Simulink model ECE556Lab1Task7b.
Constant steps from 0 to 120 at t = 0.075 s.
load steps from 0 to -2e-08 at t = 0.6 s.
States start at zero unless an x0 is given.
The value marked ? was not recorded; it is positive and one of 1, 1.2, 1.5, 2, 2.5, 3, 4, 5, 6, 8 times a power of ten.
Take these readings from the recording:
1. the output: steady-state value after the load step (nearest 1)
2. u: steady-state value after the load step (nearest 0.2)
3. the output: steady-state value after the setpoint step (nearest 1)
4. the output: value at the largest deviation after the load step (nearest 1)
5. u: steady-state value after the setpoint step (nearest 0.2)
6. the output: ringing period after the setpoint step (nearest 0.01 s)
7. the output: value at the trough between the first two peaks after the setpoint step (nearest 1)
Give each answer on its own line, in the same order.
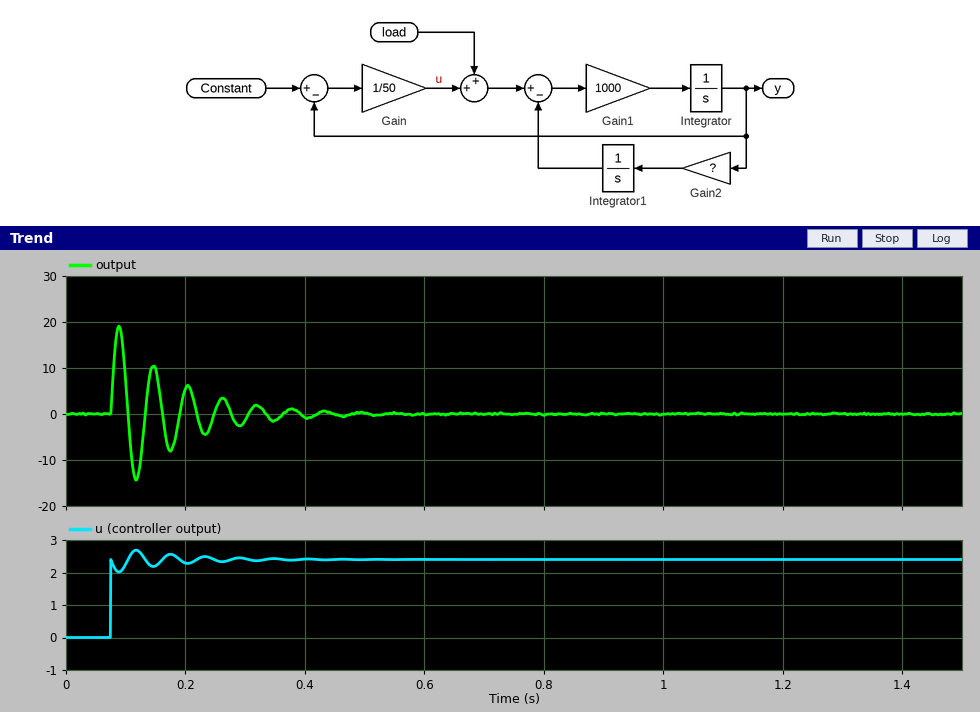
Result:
0
2.4
0
0
2.4
0.06 s
-14
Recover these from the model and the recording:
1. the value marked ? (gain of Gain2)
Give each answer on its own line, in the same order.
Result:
12
